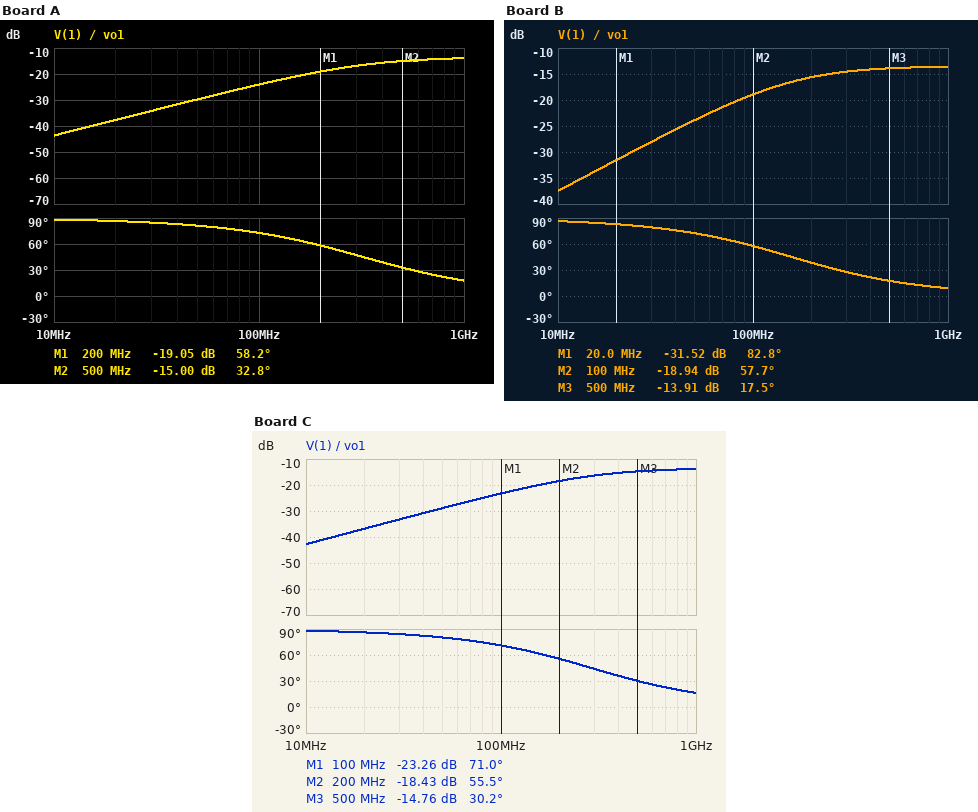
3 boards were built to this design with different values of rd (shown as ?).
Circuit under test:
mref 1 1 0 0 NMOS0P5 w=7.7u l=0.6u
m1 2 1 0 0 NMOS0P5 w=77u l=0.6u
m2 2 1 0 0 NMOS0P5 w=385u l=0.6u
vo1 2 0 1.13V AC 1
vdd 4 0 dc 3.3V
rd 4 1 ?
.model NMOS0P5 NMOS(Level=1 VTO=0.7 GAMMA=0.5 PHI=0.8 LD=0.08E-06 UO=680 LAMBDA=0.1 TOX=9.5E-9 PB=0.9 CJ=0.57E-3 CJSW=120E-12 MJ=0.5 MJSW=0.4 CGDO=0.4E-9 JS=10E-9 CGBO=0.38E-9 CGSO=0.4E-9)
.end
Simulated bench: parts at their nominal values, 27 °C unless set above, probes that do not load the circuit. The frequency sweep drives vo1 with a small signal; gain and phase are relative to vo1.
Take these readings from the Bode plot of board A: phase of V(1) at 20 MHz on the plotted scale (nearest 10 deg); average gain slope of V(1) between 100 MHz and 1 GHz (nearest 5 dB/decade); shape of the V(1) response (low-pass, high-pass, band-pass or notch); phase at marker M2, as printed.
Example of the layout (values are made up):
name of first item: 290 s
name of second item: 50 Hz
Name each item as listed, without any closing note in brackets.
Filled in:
phase of V(1) at 20 MHz on the plotted scale: 90 deg
average gain slope of V(1) between 100 MHz and 1 GHz: 10 dB/decade
shape of the V(1) response: high-pass
phase at marker M2, as printed: 32.8 deg
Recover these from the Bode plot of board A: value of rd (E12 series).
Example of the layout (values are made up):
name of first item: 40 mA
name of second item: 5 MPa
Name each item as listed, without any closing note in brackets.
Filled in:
value of rd: 8.2 kΩ
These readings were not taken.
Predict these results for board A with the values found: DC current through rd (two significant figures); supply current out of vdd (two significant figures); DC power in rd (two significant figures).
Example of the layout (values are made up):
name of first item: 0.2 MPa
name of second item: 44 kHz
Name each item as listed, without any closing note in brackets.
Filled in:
DC current through rd: 280 µA
supply current out of vdd: 280 µA
DC power in rd: 620 µW
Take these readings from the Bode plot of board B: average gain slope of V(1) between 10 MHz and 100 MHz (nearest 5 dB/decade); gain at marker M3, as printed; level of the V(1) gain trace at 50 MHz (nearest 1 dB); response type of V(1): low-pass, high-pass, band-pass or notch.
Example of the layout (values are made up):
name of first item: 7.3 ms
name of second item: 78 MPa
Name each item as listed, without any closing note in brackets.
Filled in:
average gain slope of V(1) between 10 MHz and 100 MHz: 20 dB/decade
gain at marker M3, as printed: -13.91 dB
level of the V(1) gain trace at 50 MHz: -24 dB
response type of V(1): low-pass, high-pass, band-pass or notch: high-pass
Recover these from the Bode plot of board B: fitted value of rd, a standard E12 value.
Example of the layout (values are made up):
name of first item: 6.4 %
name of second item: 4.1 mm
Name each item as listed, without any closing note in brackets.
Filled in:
fitted value of rd, a standard E12 value: 33 kΩ
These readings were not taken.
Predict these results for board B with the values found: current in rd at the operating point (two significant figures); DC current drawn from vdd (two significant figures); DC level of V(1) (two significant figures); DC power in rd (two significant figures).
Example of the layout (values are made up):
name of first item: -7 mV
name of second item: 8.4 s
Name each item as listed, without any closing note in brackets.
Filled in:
current in rd at the operating point: 73 µA
DC current drawn from vdd: 73 µA
DC level of V(1): 880 mV
DC power in rd: 180 µW
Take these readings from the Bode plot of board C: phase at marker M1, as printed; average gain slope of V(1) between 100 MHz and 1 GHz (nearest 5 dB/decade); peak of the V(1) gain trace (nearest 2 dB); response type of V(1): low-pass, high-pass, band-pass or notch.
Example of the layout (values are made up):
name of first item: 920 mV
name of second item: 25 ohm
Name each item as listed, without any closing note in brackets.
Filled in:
phase at marker M1, as printed: 71.0 deg
average gain slope of V(1) between 100 MHz and 1 GHz: 10 dB/decade
peak of the V(1) gain trace: -14 dB
response type of V(1): low-pass, high-pass, band-pass or notch: high-pass
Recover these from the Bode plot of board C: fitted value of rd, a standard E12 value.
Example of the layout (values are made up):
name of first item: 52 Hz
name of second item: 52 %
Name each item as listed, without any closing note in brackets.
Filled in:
fitted value of rd, a standard E12 value: 10 kΩ
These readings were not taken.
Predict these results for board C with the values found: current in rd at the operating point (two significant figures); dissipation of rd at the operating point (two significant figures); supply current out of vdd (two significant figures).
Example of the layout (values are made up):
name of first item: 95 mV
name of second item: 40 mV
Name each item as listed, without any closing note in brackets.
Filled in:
current in rd at the operating point: 230 µA
dissipation of rd at the operating point: 520 µW
supply current out of vdd: 230 µA
